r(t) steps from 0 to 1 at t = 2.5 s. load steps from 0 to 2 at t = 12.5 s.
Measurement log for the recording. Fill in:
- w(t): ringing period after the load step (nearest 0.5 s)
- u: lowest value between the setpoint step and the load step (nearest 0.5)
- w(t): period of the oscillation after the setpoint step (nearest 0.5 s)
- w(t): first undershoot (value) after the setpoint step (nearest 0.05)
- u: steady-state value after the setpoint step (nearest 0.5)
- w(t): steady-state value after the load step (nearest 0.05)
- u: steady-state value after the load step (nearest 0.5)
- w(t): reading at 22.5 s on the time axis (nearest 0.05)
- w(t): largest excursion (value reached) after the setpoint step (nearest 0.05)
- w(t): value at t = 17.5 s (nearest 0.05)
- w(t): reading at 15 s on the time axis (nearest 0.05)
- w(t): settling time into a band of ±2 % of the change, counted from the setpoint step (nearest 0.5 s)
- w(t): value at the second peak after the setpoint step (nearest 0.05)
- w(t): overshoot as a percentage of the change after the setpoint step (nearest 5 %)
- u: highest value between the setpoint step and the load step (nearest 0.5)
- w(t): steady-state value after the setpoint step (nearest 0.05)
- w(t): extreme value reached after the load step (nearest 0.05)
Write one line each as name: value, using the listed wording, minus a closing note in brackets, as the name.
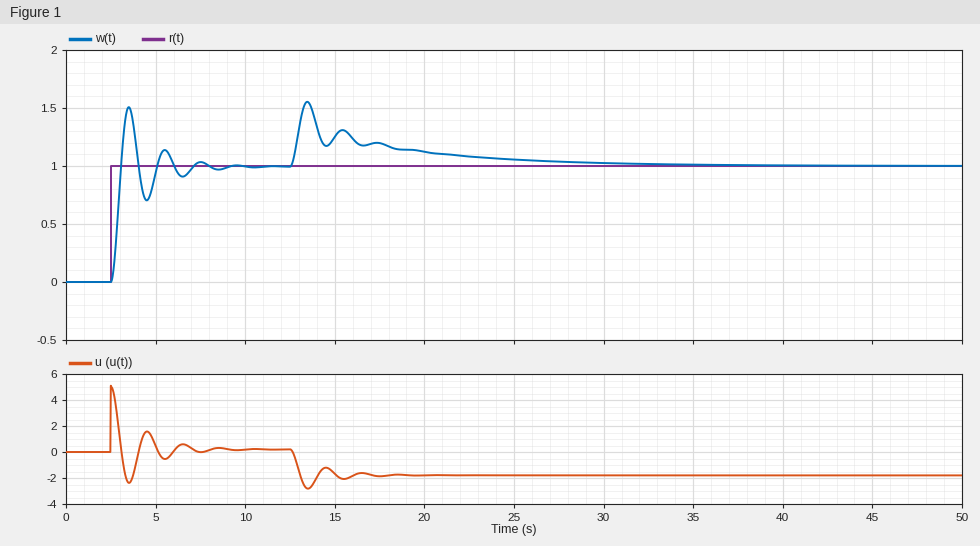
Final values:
w(t): ringing period after the load step: 2.0 s
u: lowest value between the setpoint step and the load step: -2.5
w(t): period of the oscillation after the setpoint step: 2.0 s
w(t): first undershoot (value) after the setpoint step: 0.70
u: steady-state value after the setpoint step: 0.0
w(t): steady-state value after the load step: 1.00
u: steady-state value after the load step: -2.0
w(t): reading at 22.5 s on the time axis: 1.10
w(t): largest excursion (value reached) after the setpoint step: 1.50
w(t): value at t = 17.5 s: 1.20
w(t): reading at 15 s on the time axis: 1.25
w(t): settling time into a band of ±2 % of the change, counted from the setpoint step: 6.5 s
w(t): value at the second peak after the setpoint step: 1.15
w(t): overshoot as a percentage of the change after the setpoint step: 50 %
u: highest value between the setpoint step and the load step: 5.0
w(t): steady-state value after the setpoint step: 1.00
w(t): extreme value reached after the load step: 1.55
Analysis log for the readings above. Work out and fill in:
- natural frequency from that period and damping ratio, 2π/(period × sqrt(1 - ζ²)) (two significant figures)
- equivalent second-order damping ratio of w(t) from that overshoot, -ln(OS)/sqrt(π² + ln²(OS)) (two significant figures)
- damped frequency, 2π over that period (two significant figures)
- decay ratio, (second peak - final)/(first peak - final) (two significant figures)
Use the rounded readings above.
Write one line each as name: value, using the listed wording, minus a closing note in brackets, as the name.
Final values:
natural frequency from that period and damping ratio, 2π/(period × sqrt(1 - ζ²)): 3.2 rad/s
equivalent second-order damping ratio of w(t) from that overshoot, -ln(OS)/sqrt(π² + ln²(OS)): 0.22
damped frequency, 2π over that period: 3.1 rad/s
decay ratio, (second peak - final)/(first peak - final): 0.30
